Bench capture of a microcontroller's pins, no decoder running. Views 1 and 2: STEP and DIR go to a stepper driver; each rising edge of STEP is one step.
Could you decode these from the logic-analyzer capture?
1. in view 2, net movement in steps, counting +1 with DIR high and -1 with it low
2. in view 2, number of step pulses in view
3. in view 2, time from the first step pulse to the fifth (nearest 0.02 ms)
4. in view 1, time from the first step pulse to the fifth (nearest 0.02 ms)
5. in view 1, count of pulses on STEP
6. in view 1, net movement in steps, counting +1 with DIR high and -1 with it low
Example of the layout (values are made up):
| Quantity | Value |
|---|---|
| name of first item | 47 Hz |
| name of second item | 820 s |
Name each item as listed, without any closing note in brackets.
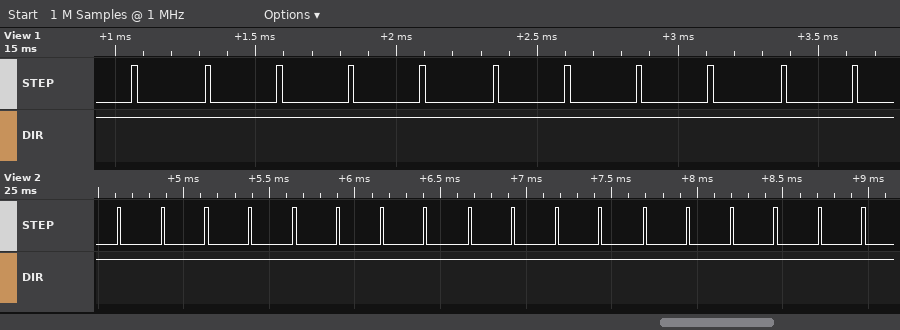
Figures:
| Quantity | Value |
|---|---|
| in view 2, net movement in steps, counting +1 with DIR high and -1 with it low | +18 |
| in view 2, number of step pulses in view | 18 |
| in view 2, time from the first step pulse to the fifth | 1.02 ms |
| in view 1, time from the first step pulse to the fifth | 1.02 ms |
| in view 1, count of pulses on STEP | 11 |
| in view 1, net movement in steps, counting +1 with DIR high and -1 with it low | +11 |
